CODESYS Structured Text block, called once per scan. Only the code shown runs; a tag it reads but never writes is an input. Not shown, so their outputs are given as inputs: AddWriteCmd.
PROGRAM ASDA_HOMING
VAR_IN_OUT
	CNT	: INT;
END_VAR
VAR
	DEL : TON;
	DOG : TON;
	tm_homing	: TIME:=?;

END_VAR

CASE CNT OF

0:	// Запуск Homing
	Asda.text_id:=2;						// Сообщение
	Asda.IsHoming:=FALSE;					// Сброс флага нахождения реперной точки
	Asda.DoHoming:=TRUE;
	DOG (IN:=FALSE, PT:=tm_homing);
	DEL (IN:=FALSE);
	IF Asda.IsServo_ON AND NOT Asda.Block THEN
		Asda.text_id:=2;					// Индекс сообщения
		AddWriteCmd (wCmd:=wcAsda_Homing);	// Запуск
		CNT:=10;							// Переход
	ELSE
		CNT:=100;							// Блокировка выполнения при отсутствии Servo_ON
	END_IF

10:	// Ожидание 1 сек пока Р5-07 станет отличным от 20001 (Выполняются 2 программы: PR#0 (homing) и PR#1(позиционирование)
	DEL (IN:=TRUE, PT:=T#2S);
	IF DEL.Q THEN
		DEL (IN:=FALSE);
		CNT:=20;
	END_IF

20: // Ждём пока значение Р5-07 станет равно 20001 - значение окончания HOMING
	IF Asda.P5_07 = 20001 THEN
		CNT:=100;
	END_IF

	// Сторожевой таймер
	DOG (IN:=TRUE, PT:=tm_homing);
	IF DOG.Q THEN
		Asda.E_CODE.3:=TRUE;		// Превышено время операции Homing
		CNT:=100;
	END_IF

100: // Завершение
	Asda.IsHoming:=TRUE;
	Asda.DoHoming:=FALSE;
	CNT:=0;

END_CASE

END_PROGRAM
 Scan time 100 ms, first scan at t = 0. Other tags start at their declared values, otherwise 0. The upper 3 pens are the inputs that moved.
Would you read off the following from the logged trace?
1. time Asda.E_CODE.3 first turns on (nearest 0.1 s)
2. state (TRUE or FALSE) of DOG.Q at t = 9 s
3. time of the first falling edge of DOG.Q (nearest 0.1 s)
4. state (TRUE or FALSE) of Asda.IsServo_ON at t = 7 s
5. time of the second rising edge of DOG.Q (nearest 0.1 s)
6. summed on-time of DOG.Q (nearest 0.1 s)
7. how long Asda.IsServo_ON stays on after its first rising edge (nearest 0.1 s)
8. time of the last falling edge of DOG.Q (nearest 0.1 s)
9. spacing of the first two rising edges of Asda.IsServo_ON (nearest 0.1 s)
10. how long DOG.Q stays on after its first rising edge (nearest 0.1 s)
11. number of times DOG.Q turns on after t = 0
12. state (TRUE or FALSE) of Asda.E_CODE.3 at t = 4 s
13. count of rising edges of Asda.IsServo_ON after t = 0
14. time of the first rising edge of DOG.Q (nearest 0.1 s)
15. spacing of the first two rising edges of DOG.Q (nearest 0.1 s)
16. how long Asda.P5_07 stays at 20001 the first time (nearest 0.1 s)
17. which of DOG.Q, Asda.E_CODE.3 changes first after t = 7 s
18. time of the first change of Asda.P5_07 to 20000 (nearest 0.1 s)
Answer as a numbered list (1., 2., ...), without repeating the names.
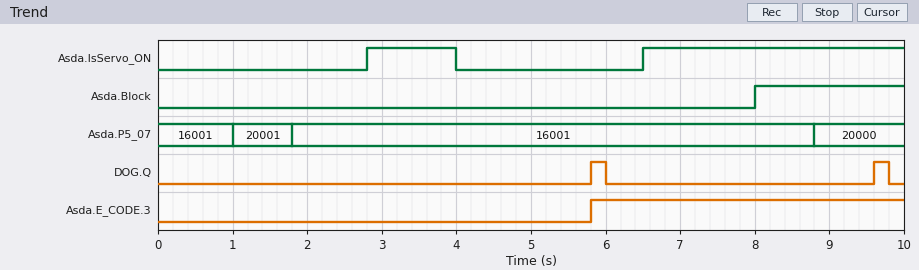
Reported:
1. 5.8 s
2. FALSE
3. 6.0 s
4. TRUE
5. 9.6 s
6. 0.4 s
7. 1.2 s
8. 9.8 s
9. 3.7 s
10. 0.2 s
11. 2
12. FALSE
13. 2
14. 5.8 s
15. 3.8 s
16. 0.8 s
17. DOG.Q
18. 8.8 s
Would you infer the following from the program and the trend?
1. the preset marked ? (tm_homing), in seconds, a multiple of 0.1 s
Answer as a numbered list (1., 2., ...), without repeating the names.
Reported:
1. 0.8 s
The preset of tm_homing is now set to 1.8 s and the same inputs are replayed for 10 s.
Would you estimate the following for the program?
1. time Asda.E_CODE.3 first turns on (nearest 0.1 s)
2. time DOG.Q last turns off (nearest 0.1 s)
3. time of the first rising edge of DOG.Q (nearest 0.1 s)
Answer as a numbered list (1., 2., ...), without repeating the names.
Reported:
1. 6.8 s
2. 7.0 s
3. 6.8 s
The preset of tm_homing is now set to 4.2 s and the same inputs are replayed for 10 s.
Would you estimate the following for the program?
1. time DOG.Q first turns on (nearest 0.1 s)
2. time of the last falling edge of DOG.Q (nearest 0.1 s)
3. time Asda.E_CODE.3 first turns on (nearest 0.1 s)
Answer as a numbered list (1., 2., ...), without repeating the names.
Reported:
1. 9.2 s
2. 9.4 s
3. 9.2 s
